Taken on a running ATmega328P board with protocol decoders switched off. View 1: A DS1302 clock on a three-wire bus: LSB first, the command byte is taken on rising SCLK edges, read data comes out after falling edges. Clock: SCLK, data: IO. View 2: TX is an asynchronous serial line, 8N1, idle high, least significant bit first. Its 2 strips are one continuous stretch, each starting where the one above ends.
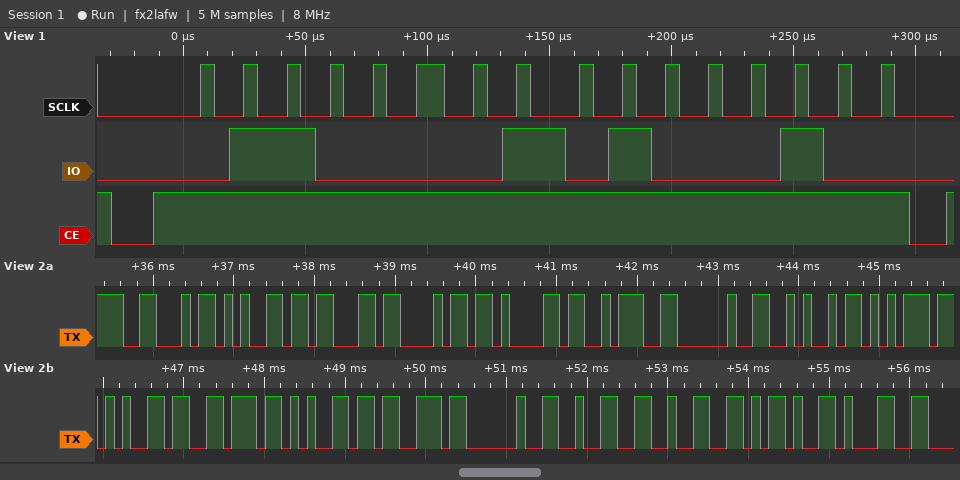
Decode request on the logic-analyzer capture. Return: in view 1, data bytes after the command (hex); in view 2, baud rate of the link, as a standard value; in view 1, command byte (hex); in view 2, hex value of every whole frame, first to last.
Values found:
22
9600 baud
0x86
46 65 63 68 61 3A 20 4A 75 65 76 65 73 20 32 32 2D 31
